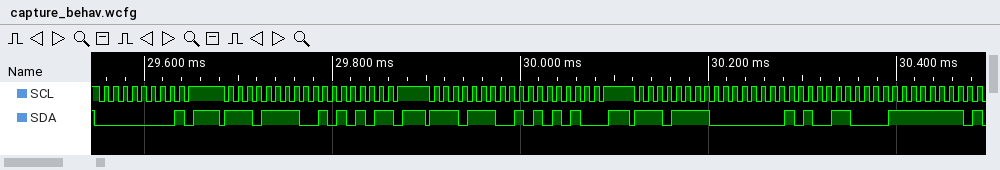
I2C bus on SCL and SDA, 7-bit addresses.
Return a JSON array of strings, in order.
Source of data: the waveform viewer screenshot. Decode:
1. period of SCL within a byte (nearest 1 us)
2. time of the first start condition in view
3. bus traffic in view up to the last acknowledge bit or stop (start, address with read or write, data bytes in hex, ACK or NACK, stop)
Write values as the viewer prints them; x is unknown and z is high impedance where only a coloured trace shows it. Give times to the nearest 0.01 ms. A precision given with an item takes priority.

["10 us", "29.55 ms", "start, address 00 write NACK, stop, start, address 77 read ACK, 55 NACK, stop, start, address 77 write ACK, AA ACK, stop, start, address 77 read ACK, 01 ACK, 98 ACK, FF ACK"]
